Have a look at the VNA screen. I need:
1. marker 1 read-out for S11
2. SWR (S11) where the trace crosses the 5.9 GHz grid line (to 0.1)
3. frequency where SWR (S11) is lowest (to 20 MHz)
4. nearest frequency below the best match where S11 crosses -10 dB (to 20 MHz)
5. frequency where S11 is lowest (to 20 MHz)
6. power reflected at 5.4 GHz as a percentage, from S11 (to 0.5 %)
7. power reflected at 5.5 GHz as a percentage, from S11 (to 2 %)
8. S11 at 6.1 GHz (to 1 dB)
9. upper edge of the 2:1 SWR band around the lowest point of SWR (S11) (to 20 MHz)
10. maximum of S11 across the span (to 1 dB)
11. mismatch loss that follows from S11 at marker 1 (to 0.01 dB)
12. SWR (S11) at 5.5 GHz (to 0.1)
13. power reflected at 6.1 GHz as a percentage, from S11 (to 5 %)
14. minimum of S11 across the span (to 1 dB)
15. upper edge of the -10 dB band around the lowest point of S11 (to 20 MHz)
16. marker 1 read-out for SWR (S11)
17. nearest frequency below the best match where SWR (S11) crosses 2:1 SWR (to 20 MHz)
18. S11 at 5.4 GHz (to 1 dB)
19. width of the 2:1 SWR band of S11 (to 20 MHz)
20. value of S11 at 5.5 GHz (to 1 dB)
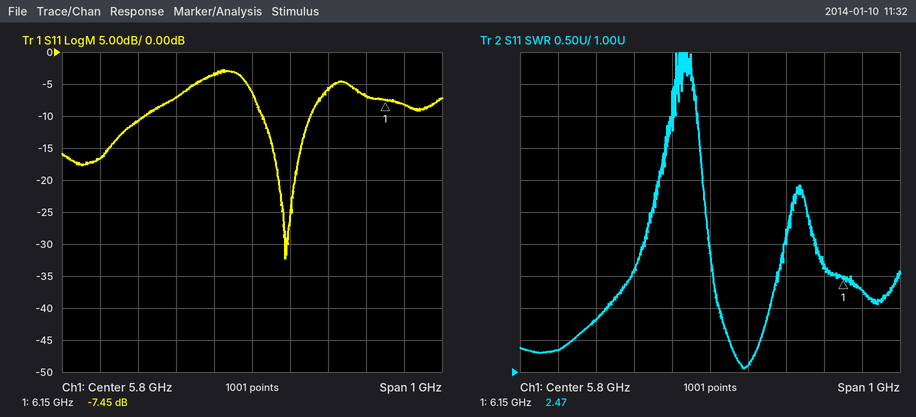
-7.45 dB
1.1
5.88 GHz
5.82 GHz
5.88 GHz
2.0 %
8 %
-7 dB
5.96 GHz
-3 dB
0.86 dB
1.8
20 %
-32 dB
5.96 GHz
2.47
5.82 GHz
-17 dB
140 MHz
-11 dB
